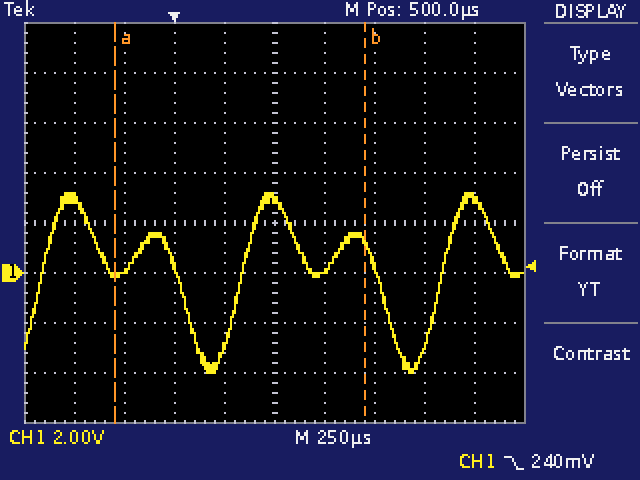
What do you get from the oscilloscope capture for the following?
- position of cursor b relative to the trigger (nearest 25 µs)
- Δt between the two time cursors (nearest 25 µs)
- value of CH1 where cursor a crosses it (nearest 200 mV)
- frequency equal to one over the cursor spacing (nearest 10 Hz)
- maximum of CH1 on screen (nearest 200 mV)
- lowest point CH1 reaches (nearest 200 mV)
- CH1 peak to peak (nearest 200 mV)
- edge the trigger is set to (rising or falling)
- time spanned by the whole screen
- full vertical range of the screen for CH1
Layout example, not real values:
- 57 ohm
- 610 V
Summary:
- +950 µs
- 1.250 ms
- 0.0 V
- 800 Hz
- 3.2 V
- -4.0 V
- 7.2 V
- falling
- 2.5 ms
- 16 V
